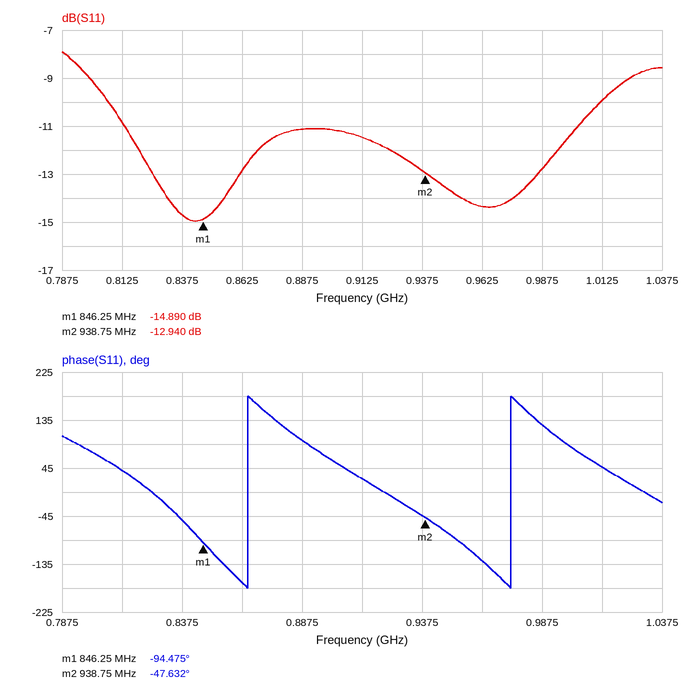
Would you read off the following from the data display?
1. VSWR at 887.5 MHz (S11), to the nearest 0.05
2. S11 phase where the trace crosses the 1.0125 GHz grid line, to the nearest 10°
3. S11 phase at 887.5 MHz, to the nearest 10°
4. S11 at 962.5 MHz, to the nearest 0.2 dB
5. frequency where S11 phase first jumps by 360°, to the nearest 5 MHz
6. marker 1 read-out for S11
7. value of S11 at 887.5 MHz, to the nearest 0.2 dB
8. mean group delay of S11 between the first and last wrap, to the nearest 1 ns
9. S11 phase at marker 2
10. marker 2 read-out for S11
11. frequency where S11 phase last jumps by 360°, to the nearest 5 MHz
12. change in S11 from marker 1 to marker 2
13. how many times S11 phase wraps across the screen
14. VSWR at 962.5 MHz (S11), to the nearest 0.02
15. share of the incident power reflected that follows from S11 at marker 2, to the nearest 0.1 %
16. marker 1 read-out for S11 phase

1.75
50°
100°
-14.4 dB
865 MHz
-14.890 dB
-11.2 dB
9 ns
-47.632°
-12.940 dB
975 MHz
1.950 dB
2
1.48
5.1 %
-94.475°
